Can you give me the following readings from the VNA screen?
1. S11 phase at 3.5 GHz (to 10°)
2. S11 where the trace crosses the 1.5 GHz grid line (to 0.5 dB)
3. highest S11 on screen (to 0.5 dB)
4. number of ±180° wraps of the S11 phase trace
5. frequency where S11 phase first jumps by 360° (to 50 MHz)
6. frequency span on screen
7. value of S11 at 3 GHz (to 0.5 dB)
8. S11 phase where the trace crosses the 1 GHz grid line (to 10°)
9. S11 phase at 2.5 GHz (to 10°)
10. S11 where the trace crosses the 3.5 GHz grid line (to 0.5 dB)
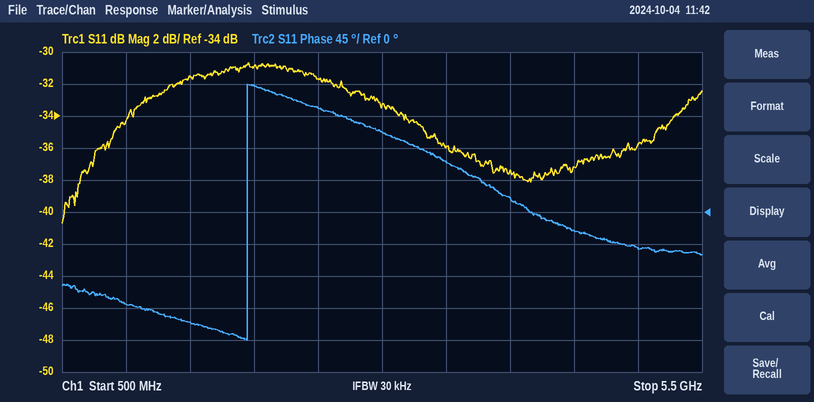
70°
-31.5 dB
-30.5 dB
1
1.95 GHz
5 GHz
-33.5 dB
-130°
150°
-36.0 dB
